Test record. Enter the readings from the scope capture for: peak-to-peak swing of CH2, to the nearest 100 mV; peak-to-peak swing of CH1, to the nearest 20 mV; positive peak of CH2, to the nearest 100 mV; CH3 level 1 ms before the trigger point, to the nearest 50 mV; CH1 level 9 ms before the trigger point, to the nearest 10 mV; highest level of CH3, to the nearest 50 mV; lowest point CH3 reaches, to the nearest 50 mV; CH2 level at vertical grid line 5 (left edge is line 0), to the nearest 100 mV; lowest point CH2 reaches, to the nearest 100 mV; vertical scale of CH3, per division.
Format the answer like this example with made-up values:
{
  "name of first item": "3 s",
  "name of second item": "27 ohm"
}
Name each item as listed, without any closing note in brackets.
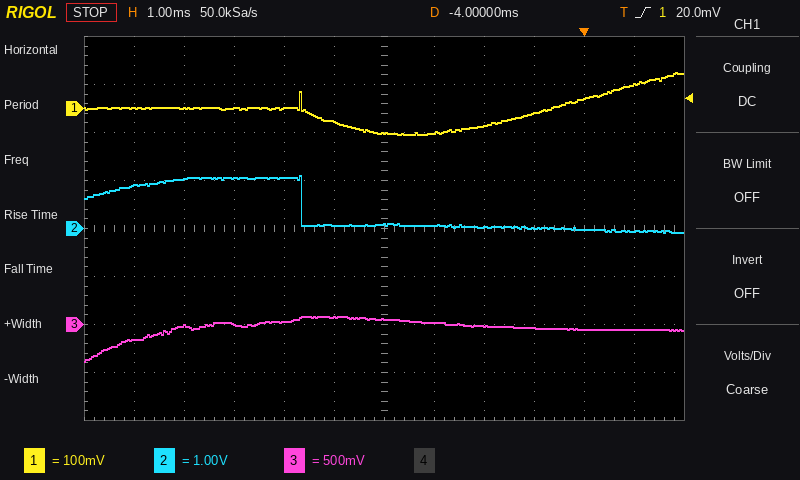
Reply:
{
  "peak-to-peak swing of CH2, to the nearest 100 mV": "1.2 V",
  "peak-to-peak swing of CH1, to the nearest 20 mV": "120 mV",
  "positive peak of CH2, to the nearest 100 mV": "1.1 V",
  "CH3 level 1 ms before the trigger point, to the nearest 50 mV": "-50 mV",
  "CH1 level 9 ms before the trigger point, to the nearest 10 mV": "0 mV",
  "highest level of CH3, to the nearest 50 mV": "100 mV",
  "lowest point CH3 reaches, to the nearest 50 mV": "-400 mV",
  "CH2 level at vertical grid line 5 (left edge is line 0), to the nearest 100 mV": "100 mV",
  "lowest point CH2 reaches, to the nearest 100 mV": "-100 mV",
  "vertical scale of CH3, per division": "500 mV"
}
